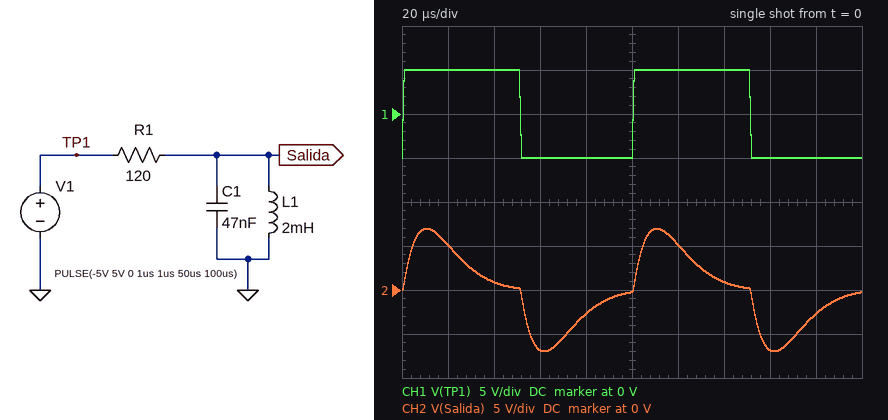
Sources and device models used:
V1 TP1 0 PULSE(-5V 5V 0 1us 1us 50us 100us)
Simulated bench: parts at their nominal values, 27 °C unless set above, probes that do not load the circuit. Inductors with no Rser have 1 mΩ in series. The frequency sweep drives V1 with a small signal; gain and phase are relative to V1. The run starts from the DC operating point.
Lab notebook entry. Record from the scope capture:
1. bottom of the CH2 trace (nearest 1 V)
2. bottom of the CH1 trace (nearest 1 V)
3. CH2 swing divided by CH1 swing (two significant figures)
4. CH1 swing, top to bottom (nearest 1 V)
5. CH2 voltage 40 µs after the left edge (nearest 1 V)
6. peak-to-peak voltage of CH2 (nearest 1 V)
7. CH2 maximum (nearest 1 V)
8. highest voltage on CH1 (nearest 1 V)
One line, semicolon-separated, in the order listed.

-7 V; -5 V; 1.4; 10 V; 1 V; 14 V; 7 V; 5 V
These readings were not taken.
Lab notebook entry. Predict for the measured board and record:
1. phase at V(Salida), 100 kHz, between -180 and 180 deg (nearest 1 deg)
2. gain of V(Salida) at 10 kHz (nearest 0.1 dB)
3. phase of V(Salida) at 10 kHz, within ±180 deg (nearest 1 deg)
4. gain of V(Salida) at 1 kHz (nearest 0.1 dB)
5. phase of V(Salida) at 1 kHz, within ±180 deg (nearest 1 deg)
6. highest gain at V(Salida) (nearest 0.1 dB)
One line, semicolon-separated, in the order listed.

-74 deg; -1.3 dB; 31 deg; -19.6 dB; 84 deg; 0 dB
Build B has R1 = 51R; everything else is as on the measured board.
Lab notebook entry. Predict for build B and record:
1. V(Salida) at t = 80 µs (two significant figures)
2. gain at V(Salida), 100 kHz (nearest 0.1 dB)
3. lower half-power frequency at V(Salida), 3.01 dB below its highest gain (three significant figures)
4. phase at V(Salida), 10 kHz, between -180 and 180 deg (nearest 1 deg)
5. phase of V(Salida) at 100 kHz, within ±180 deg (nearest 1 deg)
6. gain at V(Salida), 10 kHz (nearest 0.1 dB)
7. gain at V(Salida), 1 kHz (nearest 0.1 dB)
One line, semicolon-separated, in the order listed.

-4.0 V; -5.0 dB; 3.84 kHz; 14 deg; -56 deg; -0.3 dB; -12.4 dB
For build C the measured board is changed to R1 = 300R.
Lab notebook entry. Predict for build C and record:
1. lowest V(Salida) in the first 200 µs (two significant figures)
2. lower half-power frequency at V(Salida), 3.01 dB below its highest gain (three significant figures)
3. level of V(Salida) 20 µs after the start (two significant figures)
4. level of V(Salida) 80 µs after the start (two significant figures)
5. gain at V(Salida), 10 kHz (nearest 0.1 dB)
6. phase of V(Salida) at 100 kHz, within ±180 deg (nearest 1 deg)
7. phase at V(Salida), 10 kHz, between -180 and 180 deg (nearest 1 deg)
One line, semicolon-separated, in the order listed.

-4.6 V; 11.7 kHz; 3.5 V; -560 mV; -5.1 dB; -83 deg; 56 deg
